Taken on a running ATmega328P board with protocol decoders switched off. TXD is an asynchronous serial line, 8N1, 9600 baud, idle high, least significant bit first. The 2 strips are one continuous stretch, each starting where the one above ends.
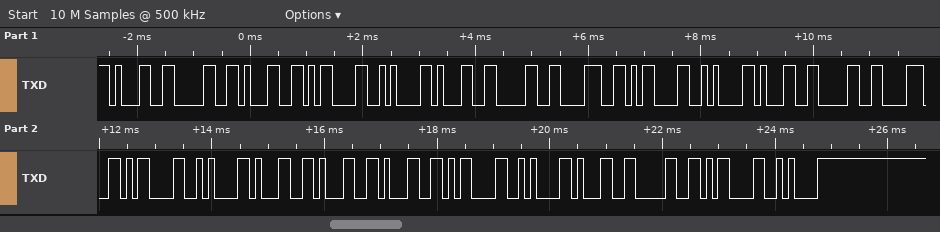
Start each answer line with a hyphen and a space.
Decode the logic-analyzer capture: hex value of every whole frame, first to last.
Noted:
- 0x31 0x30 0x31 0x0D 0x0A 0x31 0x30 0x38 0x0D 0x0A 0x31 0x30 0x38 0x0D 0x0A 0x31 0x31 0x31 0x0D 0x0A 0x31 0x30 0x0D 0x0A
